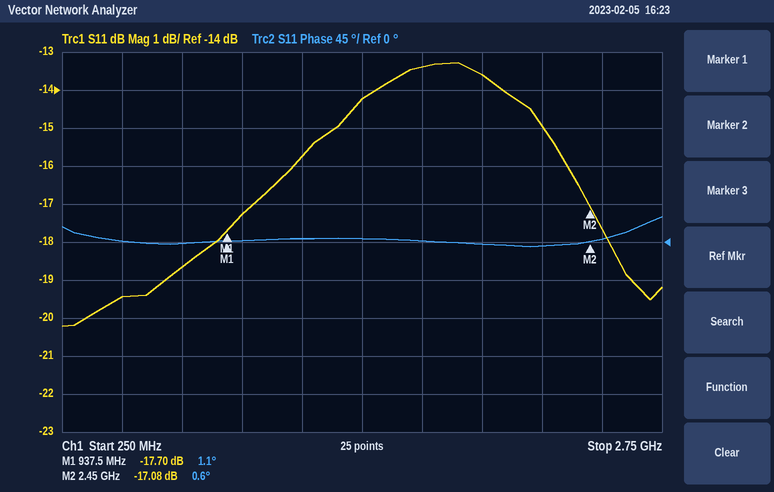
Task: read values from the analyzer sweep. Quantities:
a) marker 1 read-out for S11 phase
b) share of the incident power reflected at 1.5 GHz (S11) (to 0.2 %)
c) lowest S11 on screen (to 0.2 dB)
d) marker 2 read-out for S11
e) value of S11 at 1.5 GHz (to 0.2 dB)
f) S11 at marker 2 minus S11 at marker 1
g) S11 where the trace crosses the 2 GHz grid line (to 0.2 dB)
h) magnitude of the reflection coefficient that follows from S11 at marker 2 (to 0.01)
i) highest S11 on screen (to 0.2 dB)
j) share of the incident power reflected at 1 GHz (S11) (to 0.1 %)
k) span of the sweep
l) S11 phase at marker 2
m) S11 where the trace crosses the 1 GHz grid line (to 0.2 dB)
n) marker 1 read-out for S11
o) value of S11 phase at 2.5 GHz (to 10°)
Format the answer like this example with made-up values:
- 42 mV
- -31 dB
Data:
- 1.1°
- 3.8 %
- -20.2 dB
- -17.08 dB
- -14.2 dB
- 0.62 dB
- -13.6 dB
- 0.14
- -13.2 dB
- 1.9 %
- 2.5 GHz
- 0.6°
- -17.2 dB
- -17.70 dB
- 0°
